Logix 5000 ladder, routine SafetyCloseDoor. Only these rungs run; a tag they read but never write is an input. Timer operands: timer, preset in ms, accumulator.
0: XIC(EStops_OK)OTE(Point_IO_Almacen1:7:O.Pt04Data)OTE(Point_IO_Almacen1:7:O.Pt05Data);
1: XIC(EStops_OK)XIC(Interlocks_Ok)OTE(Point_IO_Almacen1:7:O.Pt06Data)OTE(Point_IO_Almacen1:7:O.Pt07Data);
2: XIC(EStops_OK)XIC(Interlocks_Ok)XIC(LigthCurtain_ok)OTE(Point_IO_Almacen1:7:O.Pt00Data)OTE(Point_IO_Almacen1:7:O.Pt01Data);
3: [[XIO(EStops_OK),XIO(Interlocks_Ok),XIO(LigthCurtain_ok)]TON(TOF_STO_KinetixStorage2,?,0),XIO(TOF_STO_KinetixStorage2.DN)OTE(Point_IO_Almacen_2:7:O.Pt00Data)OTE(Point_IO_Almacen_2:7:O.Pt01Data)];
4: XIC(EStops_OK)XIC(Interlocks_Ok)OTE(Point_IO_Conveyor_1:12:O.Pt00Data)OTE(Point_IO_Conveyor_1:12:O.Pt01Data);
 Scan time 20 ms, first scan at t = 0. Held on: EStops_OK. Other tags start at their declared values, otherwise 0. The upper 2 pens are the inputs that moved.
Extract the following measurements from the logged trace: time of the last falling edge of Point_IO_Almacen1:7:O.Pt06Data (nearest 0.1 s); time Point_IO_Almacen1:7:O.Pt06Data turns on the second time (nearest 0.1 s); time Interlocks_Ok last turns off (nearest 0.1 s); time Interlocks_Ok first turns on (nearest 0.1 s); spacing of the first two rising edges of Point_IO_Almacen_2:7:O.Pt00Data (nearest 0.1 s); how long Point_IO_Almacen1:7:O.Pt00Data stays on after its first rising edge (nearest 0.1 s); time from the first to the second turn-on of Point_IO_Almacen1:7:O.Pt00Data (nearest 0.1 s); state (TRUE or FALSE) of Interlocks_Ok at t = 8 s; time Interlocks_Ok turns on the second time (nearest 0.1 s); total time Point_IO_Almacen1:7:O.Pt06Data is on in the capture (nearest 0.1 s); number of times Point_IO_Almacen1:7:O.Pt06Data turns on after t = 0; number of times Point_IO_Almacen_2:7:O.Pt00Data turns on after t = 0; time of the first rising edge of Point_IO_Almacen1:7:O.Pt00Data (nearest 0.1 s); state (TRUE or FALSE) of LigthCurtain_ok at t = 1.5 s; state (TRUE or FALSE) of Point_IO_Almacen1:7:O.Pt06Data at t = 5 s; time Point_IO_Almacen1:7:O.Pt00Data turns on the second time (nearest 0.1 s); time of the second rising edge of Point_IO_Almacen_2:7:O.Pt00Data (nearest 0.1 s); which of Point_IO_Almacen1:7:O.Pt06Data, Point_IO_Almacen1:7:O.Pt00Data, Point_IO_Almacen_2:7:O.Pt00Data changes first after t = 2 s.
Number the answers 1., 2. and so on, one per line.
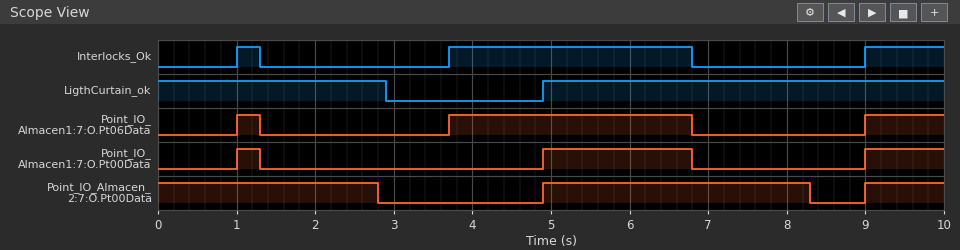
1. 6.8 s
2. 3.7 s
3. 6.8 s
4. 1.0 s
5. 4.1 s
6. 0.3 s
7. 3.9 s
8. FALSE
9. 3.7 s
10. 4.4 s
11. 3
12. 2
13. 1.0 s
14. TRUE
15. TRUE
16. 4.9 s
17. 9.0 s
18. Point_IO_Almacen_2:7:O.Pt00Data
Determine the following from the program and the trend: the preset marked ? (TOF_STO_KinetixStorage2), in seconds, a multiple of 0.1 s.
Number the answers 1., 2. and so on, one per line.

1. 1.5 s
